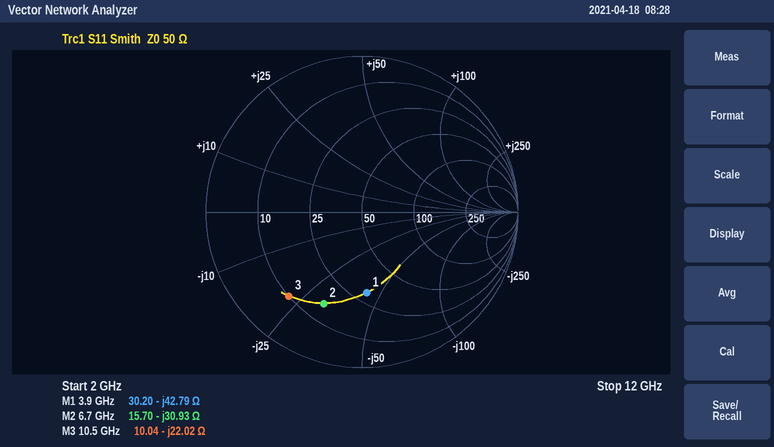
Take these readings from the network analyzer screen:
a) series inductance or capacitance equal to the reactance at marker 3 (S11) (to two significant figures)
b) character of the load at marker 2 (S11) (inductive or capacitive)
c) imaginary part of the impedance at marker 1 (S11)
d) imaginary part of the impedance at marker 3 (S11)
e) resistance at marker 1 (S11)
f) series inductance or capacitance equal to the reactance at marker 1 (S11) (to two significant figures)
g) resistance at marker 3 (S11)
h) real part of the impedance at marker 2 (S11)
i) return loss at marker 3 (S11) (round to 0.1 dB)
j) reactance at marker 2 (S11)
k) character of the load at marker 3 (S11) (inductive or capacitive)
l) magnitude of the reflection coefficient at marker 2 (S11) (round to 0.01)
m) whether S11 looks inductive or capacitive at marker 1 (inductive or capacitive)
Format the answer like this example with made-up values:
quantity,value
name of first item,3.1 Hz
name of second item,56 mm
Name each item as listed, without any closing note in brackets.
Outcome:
quantity,value
series inductance or capacitance equal to the reactance at marker 3 (S11),690 fF
character of the load at marker 2 (S11),capacitive
imaginary part of the impedance at marker 1,-42.79 Ω
imaginary part of the impedance at marker 3,-22.02 Ω
resistance at marker 1,30.20 Ω
series inductance or capacitance equal to the reactance at marker 1 (S11),950 fF
resistance at marker 3,10.04 Ω
real part of the impedance at marker 2,15.70 Ω
return loss at marker 3 (S11),2.9 dB
reactance at marker 2,-30.93 Ω
character of the load at marker 3 (S11),capacitive
magnitude of the reflection coefficient at marker 2 (S11),0.64
whether S11 looks inductive or capacitive at marker 1,capacitive
